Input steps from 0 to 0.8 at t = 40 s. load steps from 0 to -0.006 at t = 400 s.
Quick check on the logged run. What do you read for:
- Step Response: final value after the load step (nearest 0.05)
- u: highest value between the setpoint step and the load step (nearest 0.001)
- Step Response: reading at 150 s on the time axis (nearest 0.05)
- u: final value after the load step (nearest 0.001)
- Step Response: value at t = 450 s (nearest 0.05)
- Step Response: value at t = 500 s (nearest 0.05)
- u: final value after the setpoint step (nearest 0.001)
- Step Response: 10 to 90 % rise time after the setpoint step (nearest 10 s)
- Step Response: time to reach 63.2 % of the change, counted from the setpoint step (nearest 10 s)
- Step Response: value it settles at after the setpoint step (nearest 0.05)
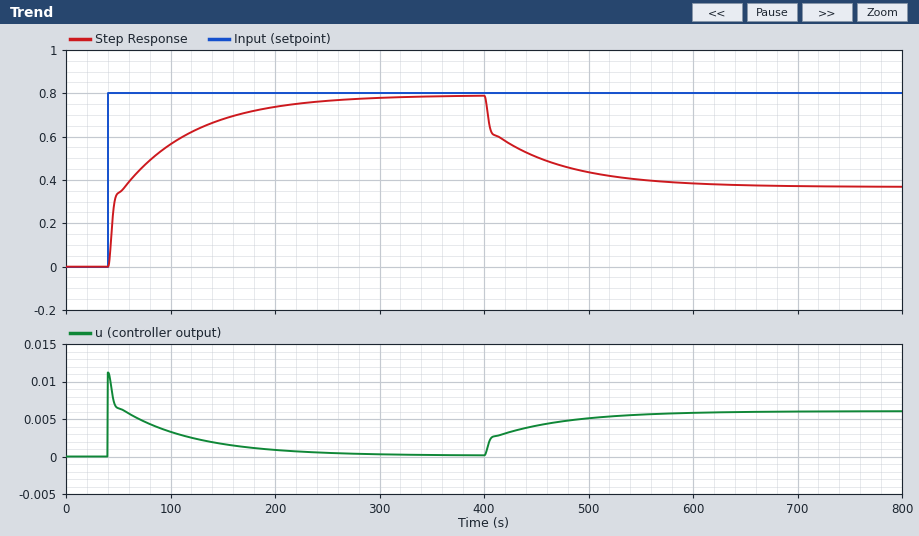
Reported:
0.35
0.011
0.70
0.006
0.50
0.45
0.000
130 s
40 s
0.80
